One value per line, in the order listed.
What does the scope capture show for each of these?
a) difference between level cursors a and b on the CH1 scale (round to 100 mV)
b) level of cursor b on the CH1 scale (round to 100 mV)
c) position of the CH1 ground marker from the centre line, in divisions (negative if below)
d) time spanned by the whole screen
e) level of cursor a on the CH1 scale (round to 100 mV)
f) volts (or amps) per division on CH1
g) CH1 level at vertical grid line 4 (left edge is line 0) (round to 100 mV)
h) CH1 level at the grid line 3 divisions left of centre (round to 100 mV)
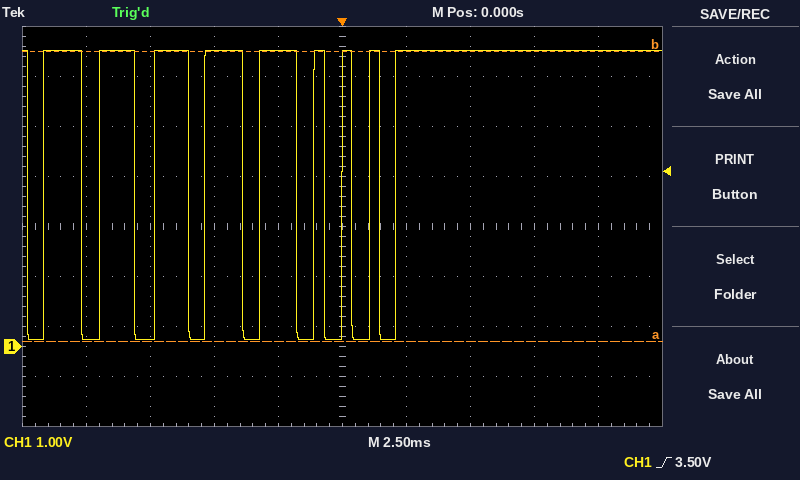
5.8 V
5.9 V
-2.4 div
25 ms
100 mV
1 V
5.9 V
100 mV
